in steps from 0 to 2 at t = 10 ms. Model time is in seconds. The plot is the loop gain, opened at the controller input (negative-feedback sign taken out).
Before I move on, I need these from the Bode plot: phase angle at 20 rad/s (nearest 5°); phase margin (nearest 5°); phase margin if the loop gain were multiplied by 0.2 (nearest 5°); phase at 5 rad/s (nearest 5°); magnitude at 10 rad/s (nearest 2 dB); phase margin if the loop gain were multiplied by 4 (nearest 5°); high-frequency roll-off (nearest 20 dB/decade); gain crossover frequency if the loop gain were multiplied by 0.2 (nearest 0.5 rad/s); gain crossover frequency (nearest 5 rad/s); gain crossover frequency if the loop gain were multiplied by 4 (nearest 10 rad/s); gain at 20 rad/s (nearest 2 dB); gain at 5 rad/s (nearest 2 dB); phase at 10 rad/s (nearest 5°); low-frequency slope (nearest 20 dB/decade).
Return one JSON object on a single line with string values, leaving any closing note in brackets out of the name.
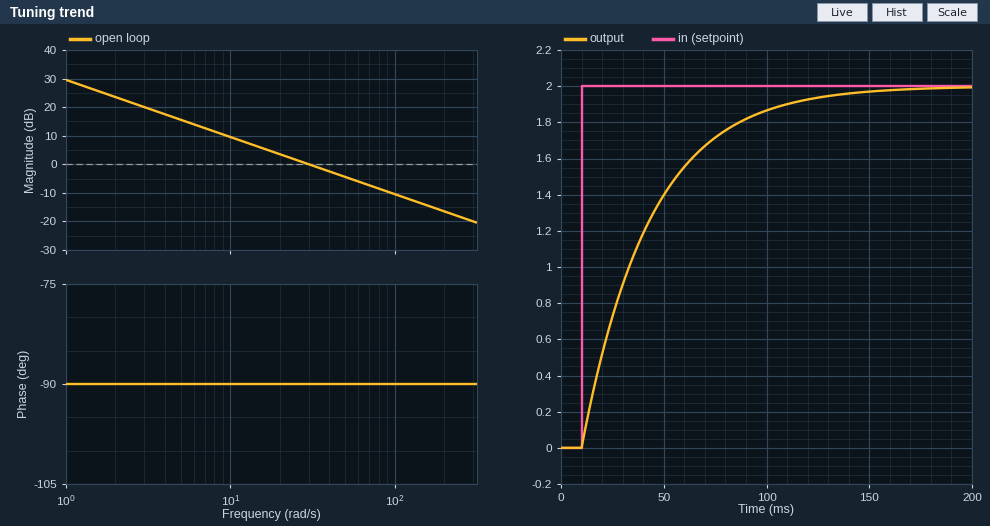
{"phase angle at 20 rad/s": "-90°", "phase margin": "90°", "phase margin if the loop gain were multiplied by 0.2": "90°", "phase at 5 rad/s": "-90°", "magnitude at 10 rad/s": "10 dB", "phase margin if the loop gain were multiplied by 4": "90°", "high-frequency roll-off": "-20 dB/decade", "gain crossover frequency if the loop gain were multiplied by 0.2": "6.0 rad/s", "gain crossover frequency": "30 rad/s", "gain crossover frequency if the loop gain were multiplied by 4": "120 rad/s", "gain at 20 rad/s": "4 dB", "gain at 5 rad/s": "16 dB", "phase at 10 rad/s": "-90°", "low-frequency slope": "-20 dB/decade"}
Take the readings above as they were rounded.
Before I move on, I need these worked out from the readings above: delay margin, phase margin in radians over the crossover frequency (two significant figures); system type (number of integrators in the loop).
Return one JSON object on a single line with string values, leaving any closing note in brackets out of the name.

{"delay margin, phase margin in radians over the crossover frequency": "0.052 s", "system type": "1"}
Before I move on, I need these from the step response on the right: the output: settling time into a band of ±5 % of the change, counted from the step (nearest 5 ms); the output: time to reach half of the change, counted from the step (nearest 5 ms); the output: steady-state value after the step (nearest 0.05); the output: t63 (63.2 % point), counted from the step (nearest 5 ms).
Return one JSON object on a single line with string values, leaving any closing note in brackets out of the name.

{"the output: settling time into a band of ±5 % of the change, counted from the step": "100 ms", "the output: time to reach half of the change, counted from the step": "25 ms", "the output: steady-state value after the step": "2.00", "the output: t63 (63.2 % point), counted from the step": "35 ms"}
